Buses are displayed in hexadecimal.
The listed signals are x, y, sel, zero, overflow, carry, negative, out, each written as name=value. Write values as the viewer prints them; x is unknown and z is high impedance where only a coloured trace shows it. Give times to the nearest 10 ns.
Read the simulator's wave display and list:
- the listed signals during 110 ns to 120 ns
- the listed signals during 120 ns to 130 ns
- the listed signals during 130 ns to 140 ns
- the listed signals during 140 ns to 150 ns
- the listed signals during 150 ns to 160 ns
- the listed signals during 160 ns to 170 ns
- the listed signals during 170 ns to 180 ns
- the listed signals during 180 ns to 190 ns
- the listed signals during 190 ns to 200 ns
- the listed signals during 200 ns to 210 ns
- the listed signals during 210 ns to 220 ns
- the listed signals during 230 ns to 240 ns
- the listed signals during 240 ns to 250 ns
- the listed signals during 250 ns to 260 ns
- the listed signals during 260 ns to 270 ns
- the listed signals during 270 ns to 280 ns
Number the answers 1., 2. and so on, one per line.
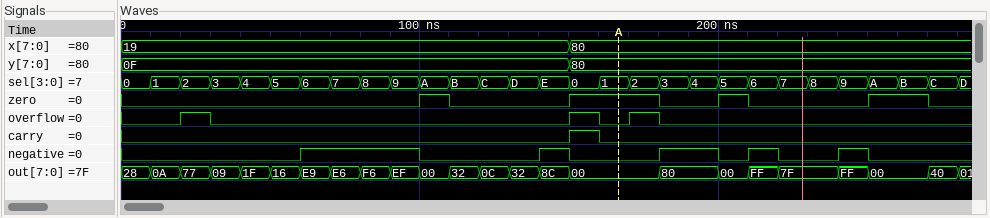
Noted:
1. x=19, y=0F, sel=B, zero=0, overflow=0, carry=0, negative=0, out=32
2. x=19, y=0F, sel=C, zero=0, overflow=0, carry=0, negative=0, out=0C
3. x=19, y=0F, sel=D, zero=0, overflow=0, carry=0, negative=0, out=32
4. x=19, y=0F, sel=E, zero=0, overflow=0, carry=0, negative=1, out=8C
5. x=80, y=80, sel=0, zero=1, overflow=1, carry=1, negative=0, out=00
6. x=80, y=80, sel=1, zero=1, overflow=0, carry=0, negative=0, out=00
7. x=80, y=80, sel=2, zero=1, overflow=1, carry=0, negative=0, out=00
8. x=80, y=80, sel=3, zero=0, overflow=0, carry=0, negative=1, out=80
9. x=80, y=80, sel=4, zero=0, overflow=0, carry=0, negative=1, out=80
10. x=80, y=80, sel=5, zero=1, overflow=0, carry=0, negative=0, out=00
11. x=80, y=80, sel=6, zero=0, overflow=0, carry=0, negative=1, out=FF
12. x=80, y=80, sel=8, zero=0, overflow=0, carry=0, negative=0, out=7F
13. x=80, y=80, sel=9, zero=0, overflow=0, carry=0, negative=1, out=FF
14. x=80, y=80, sel=A, zero=1, overflow=0, carry=0, negative=0, out=00
15. x=80, y=80, sel=B, zero=1, overflow=0, carry=0, negative=0, out=00
16. x=80, y=80, sel=C, zero=0, overflow=0, carry=0, negative=0, out=40
